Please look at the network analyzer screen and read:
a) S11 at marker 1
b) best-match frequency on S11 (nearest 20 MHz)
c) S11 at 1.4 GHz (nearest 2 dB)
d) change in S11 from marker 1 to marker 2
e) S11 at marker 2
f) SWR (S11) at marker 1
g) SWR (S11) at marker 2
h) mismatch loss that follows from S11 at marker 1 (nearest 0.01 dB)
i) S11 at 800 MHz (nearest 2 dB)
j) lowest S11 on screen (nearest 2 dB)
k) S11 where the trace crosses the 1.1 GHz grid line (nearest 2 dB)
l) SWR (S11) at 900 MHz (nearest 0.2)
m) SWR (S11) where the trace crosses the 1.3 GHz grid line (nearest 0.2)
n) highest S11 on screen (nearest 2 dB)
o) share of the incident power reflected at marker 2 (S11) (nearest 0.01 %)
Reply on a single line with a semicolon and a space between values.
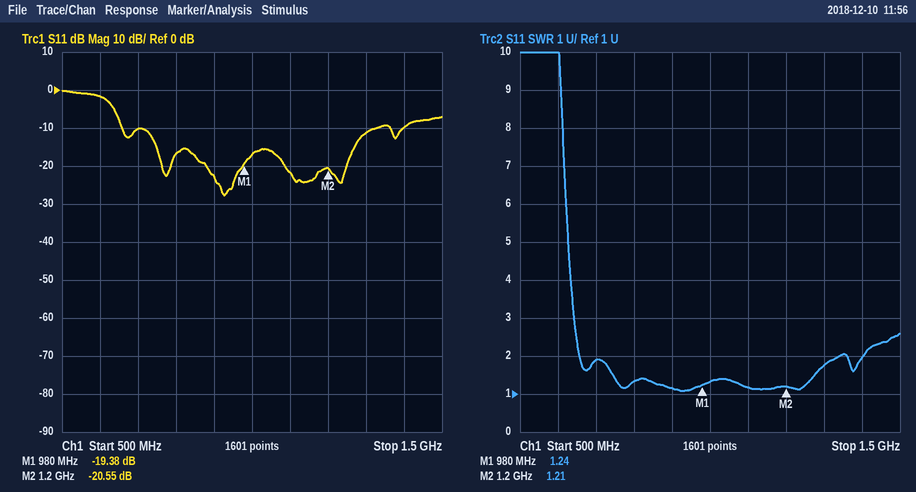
-19.38 dB; 920 MHz; -10 dB; -1.17 dB; -20.55 dB; 1.24; 1.21; 0.05 dB; -16 dB; -28 dB; -22 dB; 1.2; 1.8; 0 dB; 0.88 %
